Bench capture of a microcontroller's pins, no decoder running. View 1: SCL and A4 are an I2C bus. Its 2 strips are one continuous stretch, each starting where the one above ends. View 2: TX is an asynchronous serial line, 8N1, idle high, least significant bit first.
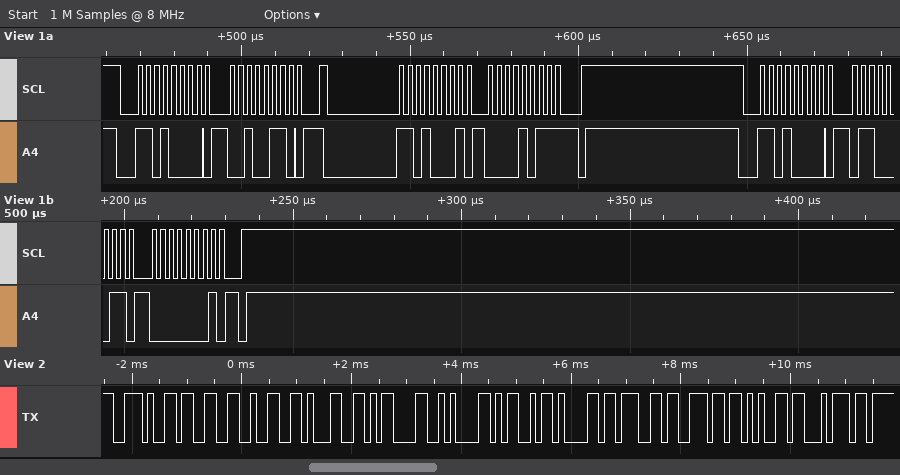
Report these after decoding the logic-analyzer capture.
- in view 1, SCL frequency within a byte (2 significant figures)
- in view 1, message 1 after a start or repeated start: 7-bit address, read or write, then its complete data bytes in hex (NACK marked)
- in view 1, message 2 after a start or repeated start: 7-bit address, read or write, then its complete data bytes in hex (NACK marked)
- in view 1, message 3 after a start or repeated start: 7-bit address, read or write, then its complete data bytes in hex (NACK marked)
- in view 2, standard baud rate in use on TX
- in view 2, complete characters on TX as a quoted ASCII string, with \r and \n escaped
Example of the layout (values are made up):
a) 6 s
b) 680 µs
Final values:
a) 400 kHz
b) 0x68 write: 26
c) 0x68 read: 0B NACK
d) 0x68 write: 63 01
e) 9600 baud
f) ".321\r\nMagnet"
